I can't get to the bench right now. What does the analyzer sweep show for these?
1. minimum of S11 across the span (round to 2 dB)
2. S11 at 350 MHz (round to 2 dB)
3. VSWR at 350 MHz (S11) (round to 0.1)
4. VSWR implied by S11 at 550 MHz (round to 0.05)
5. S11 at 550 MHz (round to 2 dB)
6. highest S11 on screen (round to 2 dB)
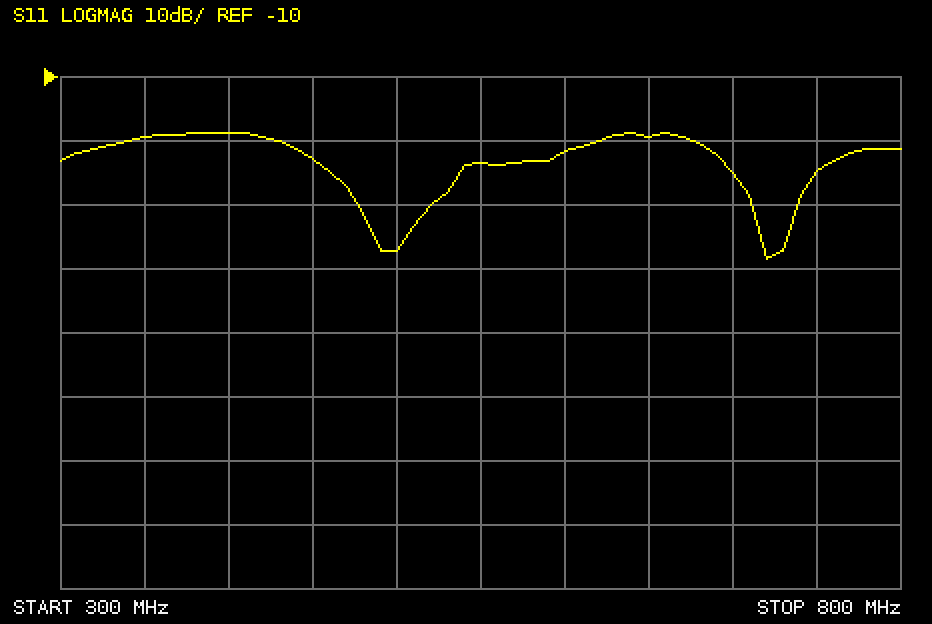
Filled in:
-38 dB
-20 dB
1.2
1.15
-24 dB
-18 dB
